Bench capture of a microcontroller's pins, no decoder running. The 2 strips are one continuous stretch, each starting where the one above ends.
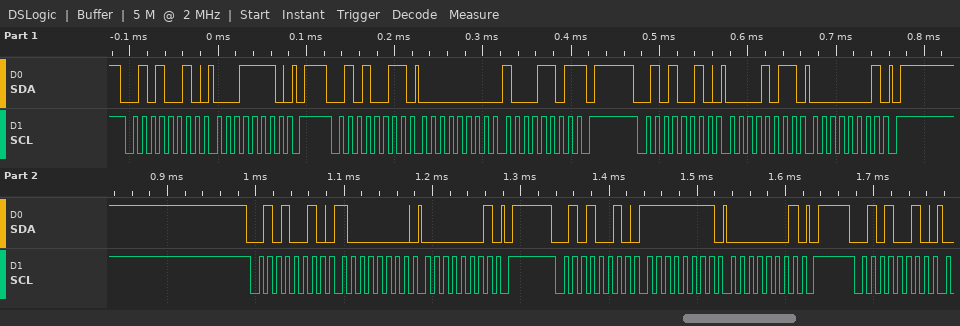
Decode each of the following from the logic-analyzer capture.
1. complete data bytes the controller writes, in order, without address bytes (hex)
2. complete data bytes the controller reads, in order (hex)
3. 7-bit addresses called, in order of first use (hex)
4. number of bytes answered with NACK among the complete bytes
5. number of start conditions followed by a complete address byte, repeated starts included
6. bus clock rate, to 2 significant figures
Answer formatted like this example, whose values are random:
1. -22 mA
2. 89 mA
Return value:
1. 1E 0B 01 80 01 FF 01
2. 00 8D
3. 0x29
4. 1
5. 6
6. 100 kHz
